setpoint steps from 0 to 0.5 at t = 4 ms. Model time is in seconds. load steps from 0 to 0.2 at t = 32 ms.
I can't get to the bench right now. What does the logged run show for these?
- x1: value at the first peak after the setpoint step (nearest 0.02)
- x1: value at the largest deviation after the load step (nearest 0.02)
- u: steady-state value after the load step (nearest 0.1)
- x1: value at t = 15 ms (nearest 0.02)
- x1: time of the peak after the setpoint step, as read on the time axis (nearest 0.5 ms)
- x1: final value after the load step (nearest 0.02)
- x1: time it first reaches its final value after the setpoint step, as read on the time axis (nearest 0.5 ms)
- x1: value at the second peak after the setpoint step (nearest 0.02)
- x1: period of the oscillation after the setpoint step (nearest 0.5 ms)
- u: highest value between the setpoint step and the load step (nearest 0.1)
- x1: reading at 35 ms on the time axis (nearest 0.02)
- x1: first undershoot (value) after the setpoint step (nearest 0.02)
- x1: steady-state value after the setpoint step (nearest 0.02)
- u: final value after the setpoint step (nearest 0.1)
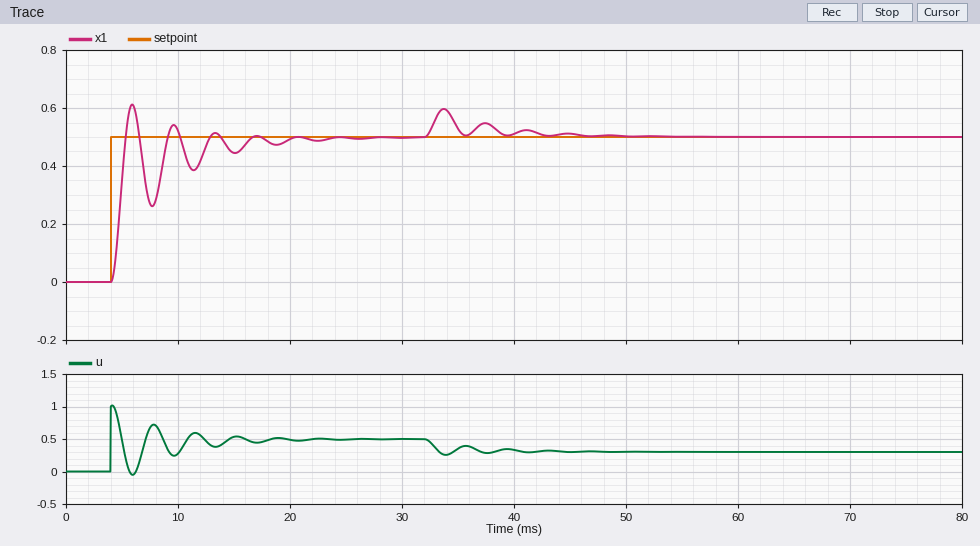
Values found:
0.62
0.60
0.3
0.44
6.0 ms
0.50
5.5 ms
0.54
3.5 ms
1.0
0.52
0.26
0.50
0.5
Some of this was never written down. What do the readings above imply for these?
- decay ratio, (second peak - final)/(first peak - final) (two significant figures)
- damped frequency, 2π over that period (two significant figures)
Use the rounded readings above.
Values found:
0.33
1.8 rad/ms
